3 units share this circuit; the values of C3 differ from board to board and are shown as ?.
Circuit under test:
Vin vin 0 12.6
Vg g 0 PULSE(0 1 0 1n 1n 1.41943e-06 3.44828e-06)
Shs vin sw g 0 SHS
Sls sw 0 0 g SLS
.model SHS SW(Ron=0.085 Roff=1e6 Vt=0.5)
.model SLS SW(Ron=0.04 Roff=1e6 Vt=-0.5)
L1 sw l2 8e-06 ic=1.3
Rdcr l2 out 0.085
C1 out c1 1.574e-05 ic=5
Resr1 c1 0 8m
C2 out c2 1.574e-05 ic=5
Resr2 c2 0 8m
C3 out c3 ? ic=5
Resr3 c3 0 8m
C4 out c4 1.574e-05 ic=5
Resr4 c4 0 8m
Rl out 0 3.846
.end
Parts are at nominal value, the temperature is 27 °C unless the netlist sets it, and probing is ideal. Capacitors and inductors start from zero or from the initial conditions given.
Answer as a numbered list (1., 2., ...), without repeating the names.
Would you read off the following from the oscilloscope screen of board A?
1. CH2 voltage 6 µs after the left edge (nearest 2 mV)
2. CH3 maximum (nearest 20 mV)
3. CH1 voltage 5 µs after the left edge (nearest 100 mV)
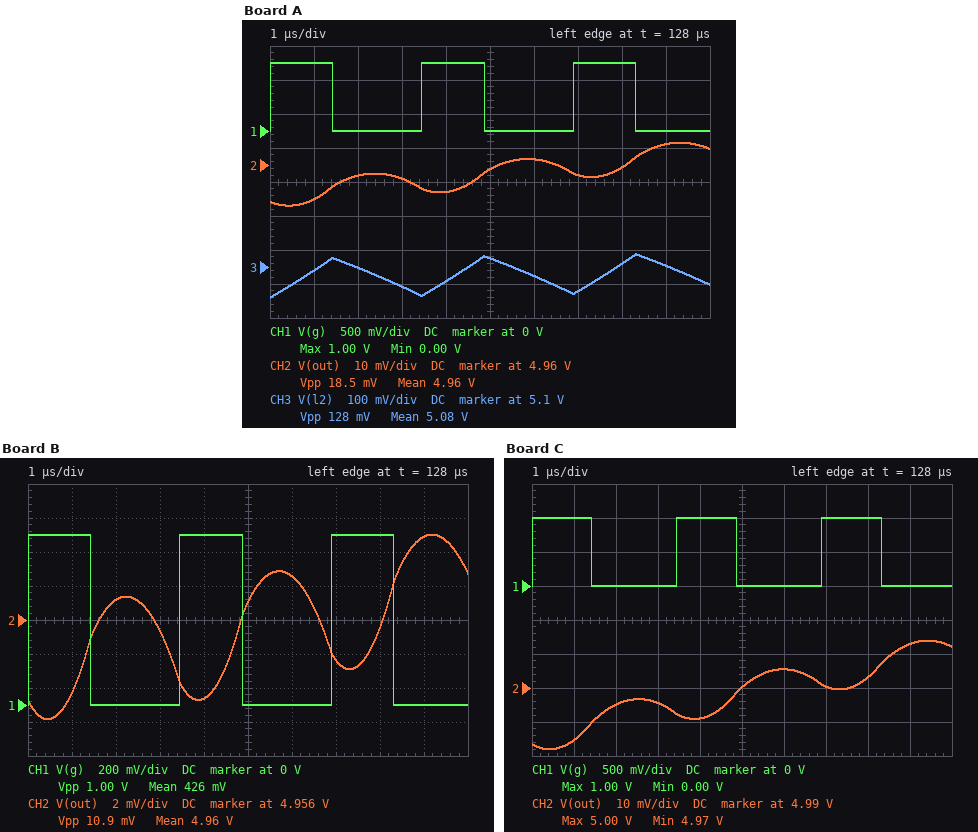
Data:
1. 4.962 V
2. 5.14 V
3. 0 V
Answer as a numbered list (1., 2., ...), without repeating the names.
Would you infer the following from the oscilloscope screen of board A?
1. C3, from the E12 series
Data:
1. 33 µF
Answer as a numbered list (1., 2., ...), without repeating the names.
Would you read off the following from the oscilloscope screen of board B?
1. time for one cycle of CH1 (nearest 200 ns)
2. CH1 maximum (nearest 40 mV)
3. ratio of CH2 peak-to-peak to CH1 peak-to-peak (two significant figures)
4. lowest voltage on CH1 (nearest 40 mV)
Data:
1. 3.4 µs
2. 1.00 V
3. 0.011
4. 0 V
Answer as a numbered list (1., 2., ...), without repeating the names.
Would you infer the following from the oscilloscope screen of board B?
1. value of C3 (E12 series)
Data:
1. 47 µF
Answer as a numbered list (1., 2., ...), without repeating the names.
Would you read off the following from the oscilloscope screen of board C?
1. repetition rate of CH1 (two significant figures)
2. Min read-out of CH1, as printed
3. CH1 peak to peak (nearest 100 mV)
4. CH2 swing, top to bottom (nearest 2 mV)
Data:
1. 290 kHz
2. 0.00 V
3. 1.0 V
4. 32 mV
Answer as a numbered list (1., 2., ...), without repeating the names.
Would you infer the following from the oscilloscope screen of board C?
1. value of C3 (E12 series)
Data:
1. 12 µF
